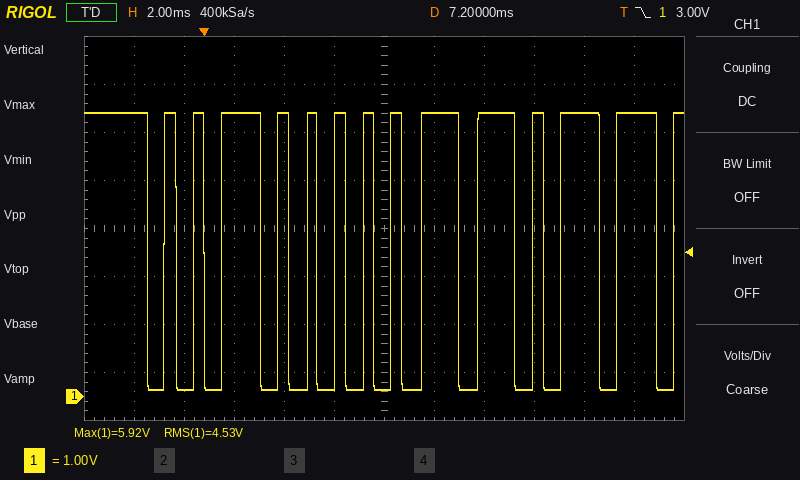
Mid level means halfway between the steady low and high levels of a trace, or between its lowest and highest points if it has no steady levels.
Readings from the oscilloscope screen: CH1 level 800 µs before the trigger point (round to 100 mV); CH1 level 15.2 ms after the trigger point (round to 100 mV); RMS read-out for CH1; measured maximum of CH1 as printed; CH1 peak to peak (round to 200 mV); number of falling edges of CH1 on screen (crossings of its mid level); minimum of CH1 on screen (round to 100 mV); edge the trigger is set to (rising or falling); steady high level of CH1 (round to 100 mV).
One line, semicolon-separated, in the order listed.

100 mV; 5.9 V; 4.53 V; 5.92 V; 5.8 V; 14; 100 mV; falling; 5.9 V
